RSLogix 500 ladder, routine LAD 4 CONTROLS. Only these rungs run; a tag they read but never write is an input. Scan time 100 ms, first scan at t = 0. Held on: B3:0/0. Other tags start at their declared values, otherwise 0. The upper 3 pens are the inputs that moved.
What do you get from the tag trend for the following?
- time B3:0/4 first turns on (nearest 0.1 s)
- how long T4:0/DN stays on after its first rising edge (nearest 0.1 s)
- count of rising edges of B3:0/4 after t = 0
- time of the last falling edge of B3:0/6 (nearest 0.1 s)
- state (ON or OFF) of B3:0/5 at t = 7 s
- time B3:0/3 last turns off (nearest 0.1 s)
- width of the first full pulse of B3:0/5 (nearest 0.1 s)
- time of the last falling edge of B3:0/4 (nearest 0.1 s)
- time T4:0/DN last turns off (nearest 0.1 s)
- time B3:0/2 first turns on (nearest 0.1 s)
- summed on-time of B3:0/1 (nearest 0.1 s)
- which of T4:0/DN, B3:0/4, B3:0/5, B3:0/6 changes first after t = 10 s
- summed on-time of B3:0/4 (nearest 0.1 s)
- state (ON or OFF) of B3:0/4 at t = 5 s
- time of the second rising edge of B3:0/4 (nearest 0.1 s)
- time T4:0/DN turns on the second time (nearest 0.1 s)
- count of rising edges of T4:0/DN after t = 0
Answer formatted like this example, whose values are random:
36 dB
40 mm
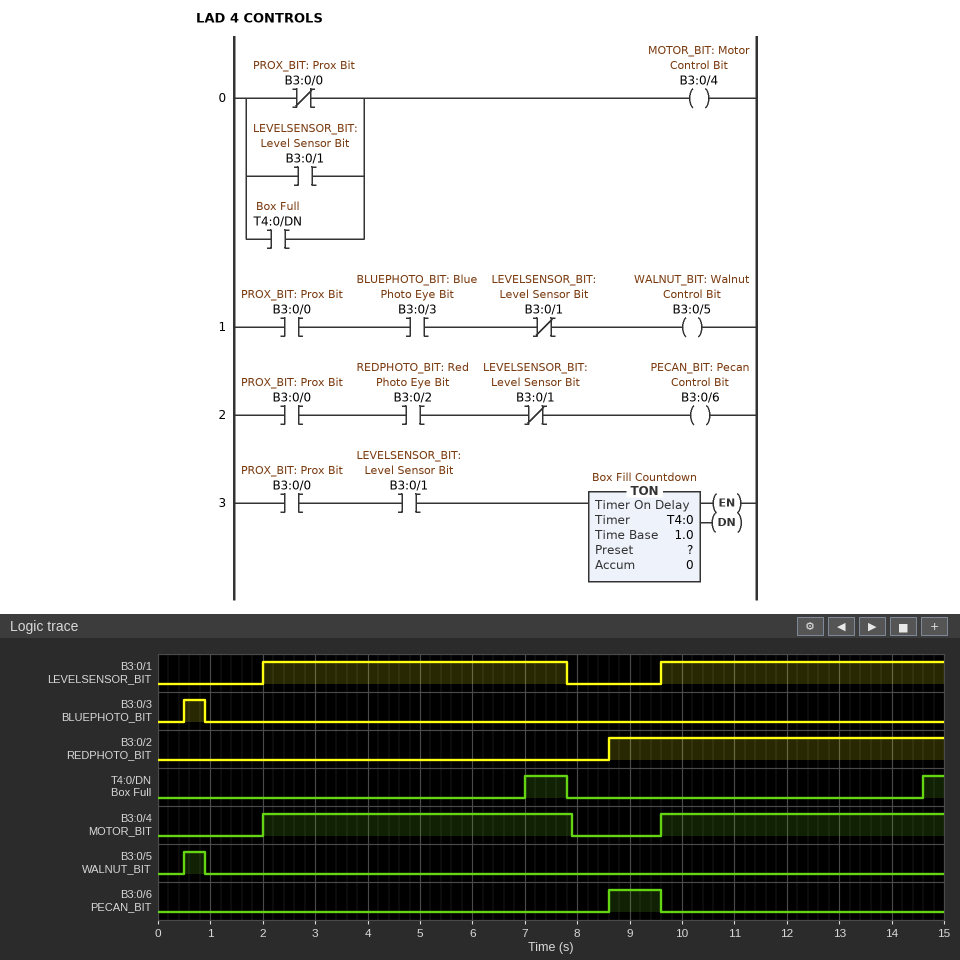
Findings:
2.0 s
0.8 s
2
9.6 s
OFF
0.9 s
0.4 s
7.9 s
7.8 s
8.6 s
11.2 s
T4:0/DN
11.3 s
ON
9.6 s
14.6 s
2
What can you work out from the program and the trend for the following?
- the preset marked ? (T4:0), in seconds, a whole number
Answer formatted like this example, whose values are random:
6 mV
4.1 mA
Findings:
5 s
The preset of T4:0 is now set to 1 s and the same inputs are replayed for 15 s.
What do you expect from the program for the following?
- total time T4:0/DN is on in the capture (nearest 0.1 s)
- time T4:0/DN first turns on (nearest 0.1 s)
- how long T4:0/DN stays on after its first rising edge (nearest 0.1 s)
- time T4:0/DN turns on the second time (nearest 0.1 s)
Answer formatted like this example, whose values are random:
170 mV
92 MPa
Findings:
9.2 s
3.0 s
4.8 s
10.6 s
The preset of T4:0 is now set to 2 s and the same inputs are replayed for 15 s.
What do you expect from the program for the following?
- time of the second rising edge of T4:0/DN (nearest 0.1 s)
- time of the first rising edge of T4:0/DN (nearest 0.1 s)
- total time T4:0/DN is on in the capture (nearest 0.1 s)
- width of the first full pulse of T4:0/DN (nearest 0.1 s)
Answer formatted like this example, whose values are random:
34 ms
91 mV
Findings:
11.6 s
4.0 s
7.2 s
3.8 s
